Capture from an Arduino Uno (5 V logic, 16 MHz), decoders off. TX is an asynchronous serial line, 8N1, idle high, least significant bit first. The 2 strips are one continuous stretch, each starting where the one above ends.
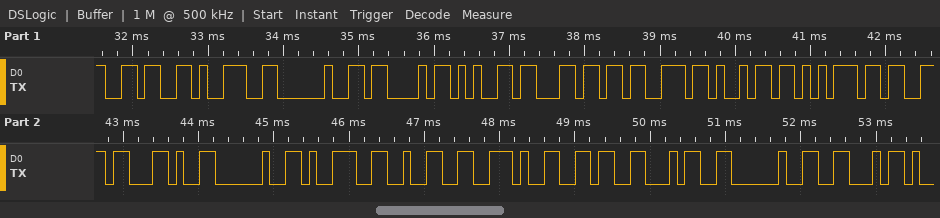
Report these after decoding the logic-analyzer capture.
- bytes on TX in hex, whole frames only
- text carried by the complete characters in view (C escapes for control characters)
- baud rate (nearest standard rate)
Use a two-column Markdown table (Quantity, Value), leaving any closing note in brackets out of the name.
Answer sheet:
| Quantity | Value |
|---|---|
| bytes on TX in hex, whole frames only | 36 39 20 43 65 6C 73 69 75 73 2C 20 39 32 2E 36 34 20 46 |
| text carried by the complete characters in view | "69 Celsius, 92.64 F" |
| baud rate | 9600 baud |
